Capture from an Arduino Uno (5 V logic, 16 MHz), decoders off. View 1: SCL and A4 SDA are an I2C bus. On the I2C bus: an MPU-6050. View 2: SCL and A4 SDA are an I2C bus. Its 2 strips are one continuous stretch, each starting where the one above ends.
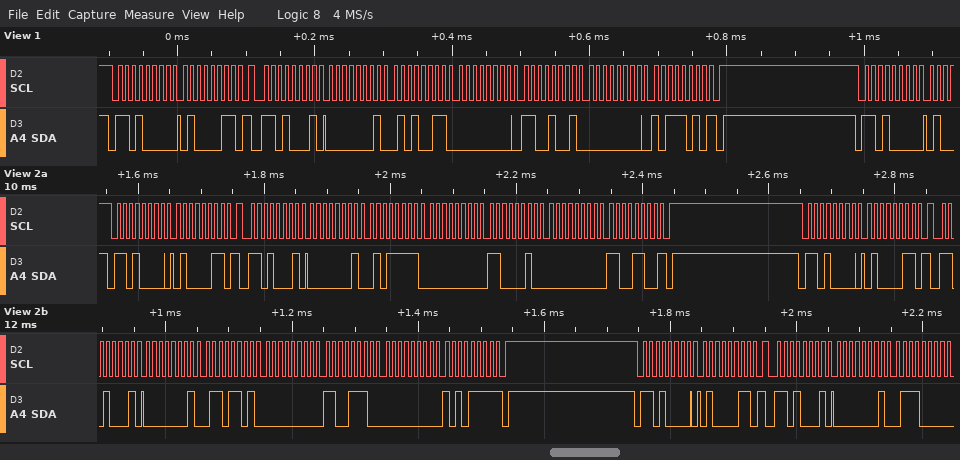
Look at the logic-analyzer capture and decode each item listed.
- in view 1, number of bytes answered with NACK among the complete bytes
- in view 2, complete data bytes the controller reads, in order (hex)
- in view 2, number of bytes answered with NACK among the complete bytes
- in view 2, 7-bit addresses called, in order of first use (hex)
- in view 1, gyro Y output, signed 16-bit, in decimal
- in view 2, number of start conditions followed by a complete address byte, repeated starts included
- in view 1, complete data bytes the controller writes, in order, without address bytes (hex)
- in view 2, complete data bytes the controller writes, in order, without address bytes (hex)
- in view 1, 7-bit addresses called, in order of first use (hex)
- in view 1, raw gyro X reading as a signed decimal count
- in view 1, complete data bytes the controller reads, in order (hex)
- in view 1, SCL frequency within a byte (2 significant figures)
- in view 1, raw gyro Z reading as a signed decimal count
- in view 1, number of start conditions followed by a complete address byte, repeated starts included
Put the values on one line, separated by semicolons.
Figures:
1; 01 5F 00 C2 00 CC 01 6D 00 CE 00 AF 01 70; 2; 0x68; 201; 6; 43; 43 43 43; 0x68; 339; 01 53 00 C9 00 BA; 100 kHz; 186; 3
